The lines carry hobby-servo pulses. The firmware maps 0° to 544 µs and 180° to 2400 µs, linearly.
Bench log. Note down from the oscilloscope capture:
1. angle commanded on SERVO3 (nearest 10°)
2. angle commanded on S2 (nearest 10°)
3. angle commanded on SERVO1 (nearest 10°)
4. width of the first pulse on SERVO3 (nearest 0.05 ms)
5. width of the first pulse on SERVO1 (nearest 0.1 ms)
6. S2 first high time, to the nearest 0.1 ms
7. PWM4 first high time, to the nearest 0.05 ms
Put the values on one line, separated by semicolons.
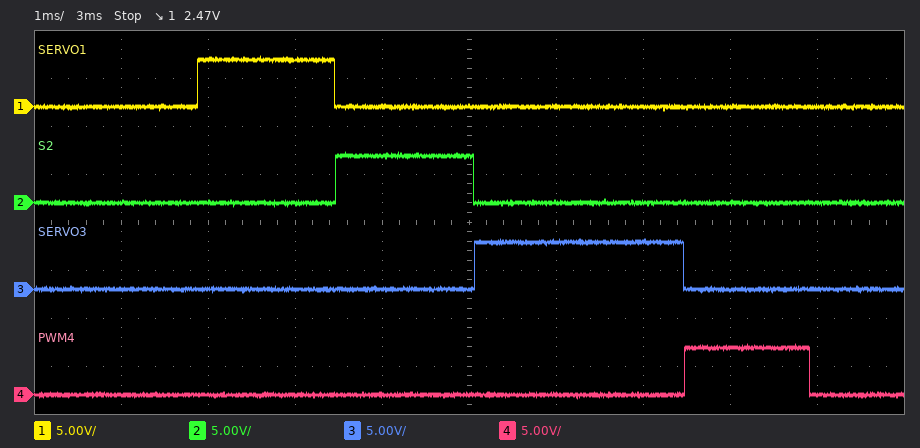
180°; 100°; 100°; 2.40 ms; 1.6 ms; 1.6 ms; 1.45 ms
